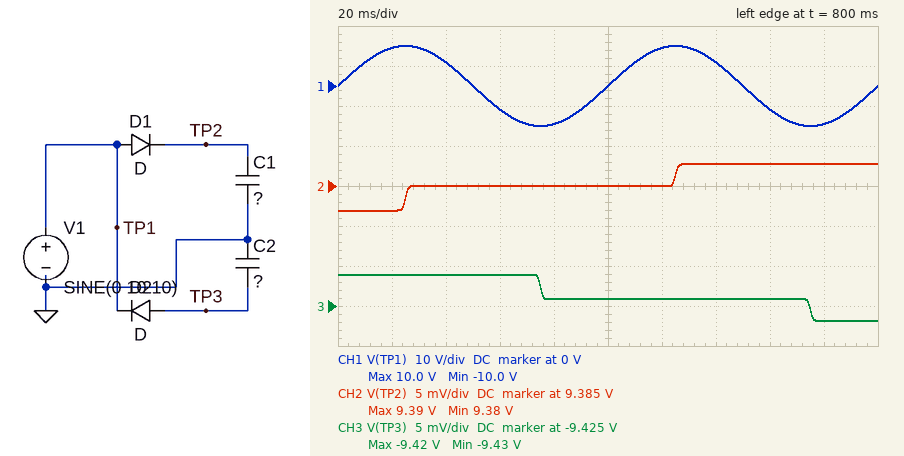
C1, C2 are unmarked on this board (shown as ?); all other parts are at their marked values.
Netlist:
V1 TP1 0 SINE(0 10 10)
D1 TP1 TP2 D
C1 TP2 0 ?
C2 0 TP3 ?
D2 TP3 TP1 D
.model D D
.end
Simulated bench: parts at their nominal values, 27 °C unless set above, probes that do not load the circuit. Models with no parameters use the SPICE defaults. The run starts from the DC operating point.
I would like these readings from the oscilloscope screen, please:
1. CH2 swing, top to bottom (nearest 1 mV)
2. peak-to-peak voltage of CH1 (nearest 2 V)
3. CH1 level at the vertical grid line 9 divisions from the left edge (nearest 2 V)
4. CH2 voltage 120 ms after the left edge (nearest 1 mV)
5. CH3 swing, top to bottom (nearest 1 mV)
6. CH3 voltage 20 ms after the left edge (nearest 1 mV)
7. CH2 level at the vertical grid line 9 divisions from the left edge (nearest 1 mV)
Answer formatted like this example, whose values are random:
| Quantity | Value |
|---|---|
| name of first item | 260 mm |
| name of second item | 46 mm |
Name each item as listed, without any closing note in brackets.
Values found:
| Quantity | Value |
|---|---|
| CH2 swing, top to bottom | 6 mV |
| peak-to-peak voltage of CH1 | 20 V |
| CH1 level at the vertical grid line 9 divisions from the left edge | -10 V |
| CH2 voltage 120 ms after the left edge | 9.385 V |
| CH3 swing, top to bottom | 6 mV |
| CH3 voltage 20 ms after the left edge | -9.421 V |
| CH2 level at the vertical grid line 9 divisions from the left edge | 9.388 V |
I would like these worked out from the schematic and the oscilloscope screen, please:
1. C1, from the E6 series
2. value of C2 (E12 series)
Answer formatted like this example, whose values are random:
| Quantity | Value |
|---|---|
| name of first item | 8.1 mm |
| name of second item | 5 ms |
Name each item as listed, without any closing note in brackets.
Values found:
| Quantity | Value |
|---|---|
| C1, from the E6 series | 150 µF |
| value of C2 | 33 µF |
